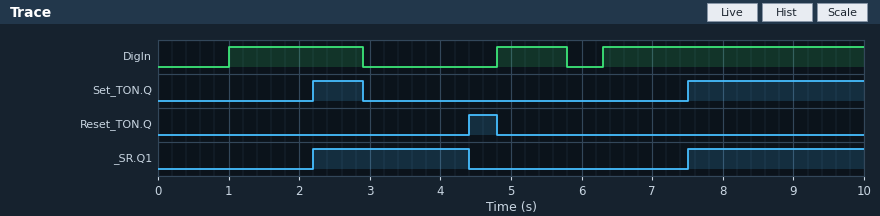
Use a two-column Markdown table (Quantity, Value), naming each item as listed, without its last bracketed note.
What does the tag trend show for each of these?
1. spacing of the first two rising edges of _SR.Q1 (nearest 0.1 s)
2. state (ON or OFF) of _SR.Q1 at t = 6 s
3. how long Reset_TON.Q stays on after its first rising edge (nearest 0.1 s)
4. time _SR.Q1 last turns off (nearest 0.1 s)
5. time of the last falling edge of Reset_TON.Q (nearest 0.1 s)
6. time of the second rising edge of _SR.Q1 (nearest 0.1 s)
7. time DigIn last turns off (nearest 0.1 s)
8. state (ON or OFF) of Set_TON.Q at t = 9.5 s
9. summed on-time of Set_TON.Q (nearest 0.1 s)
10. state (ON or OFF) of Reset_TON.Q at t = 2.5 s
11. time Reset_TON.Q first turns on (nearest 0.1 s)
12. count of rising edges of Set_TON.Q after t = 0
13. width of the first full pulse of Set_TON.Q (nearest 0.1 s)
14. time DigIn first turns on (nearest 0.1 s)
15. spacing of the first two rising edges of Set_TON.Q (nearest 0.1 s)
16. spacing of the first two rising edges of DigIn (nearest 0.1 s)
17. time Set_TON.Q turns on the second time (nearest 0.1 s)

| Quantity | Value |
|---|---|
| spacing of the first two rising edges of _SR.Q1 | 5.3 s |
| state (ON or OFF) of _SR.Q1 at t = 6 s | OFF |
| how long Reset_TON.Q stays on after its first rising edge | 0.4 s |
| time _SR.Q1 last turns off | 4.4 s |
| time of the last falling edge of Reset_TON.Q | 4.8 s |
| time of the second rising edge of _SR.Q1 | 7.5 s |
| time DigIn last turns off | 5.8 s |
| state (ON or OFF) of Set_TON.Q at t = 9.5 s | ON |
| summed on-time of Set_TON.Q | 3.2 s |
| state (ON or OFF) of Reset_TON.Q at t = 2.5 s | OFF |
| time Reset_TON.Q first turns on | 4.4 s |
| count of rising edges of Set_TON.Q after t = 0 | 2 |
| width of the first full pulse of Set_TON.Q | 0.7 s |
| time DigIn first turns on | 1.0 s |
| spacing of the first two rising edges of Set_TON.Q | 5.3 s |
| spacing of the first two rising edges of DigIn | 3.8 s |
| time Set_TON.Q turns on the second time | 7.5 s |
